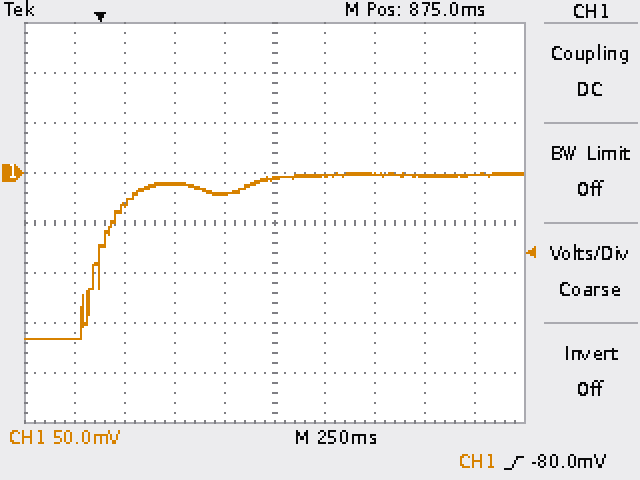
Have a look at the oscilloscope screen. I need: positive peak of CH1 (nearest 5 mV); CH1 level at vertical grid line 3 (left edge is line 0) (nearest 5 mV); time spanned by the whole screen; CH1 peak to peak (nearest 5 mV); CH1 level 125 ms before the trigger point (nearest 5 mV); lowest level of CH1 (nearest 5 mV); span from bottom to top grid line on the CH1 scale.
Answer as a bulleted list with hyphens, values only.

- 0 mV
- -10 mV
- 2.5 s
- 165 mV
- -165 mV
- -165 mV
- 400 mV
